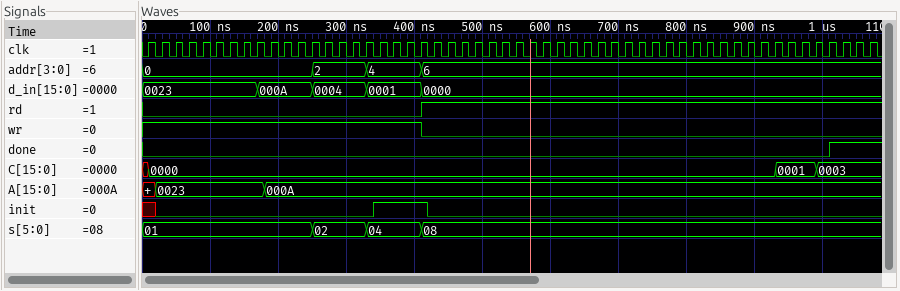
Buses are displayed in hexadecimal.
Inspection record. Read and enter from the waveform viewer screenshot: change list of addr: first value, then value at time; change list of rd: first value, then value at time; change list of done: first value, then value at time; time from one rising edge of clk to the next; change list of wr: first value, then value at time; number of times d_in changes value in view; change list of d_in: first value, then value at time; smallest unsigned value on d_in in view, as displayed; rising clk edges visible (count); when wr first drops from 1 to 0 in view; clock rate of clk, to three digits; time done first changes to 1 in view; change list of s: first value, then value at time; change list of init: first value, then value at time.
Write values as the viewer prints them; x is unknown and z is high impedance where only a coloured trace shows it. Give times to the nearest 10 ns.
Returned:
0, 2 at 250 ns, 4 at 330 ns, 6 at 410 ns
0, 1 at 410 ns
0, 1 at 1010 ns
20 ns
1, 0 at 410 ns
4
0023, 000A at 170 ns, 0004 at 250 ns, 0001 at 330 ns, 0000 at 410 ns
0000
54
410 ns
50.0 MHz
1010 ns
01, 02 at 250 ns, 04 at 330 ns, 08 at 410 ns
x, 0 at 20 ns, 1 at 340 ns, 0 at 420 ns
